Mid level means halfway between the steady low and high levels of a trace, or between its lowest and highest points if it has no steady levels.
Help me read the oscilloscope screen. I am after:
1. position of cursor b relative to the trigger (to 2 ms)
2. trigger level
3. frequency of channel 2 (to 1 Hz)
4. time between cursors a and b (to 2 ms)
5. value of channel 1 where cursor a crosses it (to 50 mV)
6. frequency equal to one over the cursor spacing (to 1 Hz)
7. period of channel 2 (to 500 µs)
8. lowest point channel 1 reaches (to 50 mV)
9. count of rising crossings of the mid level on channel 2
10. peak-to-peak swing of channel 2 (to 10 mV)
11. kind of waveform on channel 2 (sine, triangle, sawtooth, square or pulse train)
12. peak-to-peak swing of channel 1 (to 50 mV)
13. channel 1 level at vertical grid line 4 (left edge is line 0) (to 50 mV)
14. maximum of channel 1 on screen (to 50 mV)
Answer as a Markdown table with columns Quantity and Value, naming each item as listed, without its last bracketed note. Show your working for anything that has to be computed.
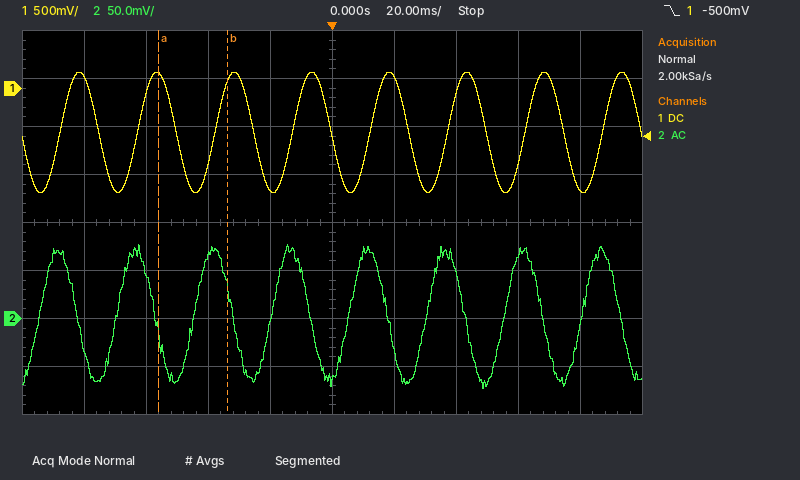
| Quantity | Value |
|---|---|
| position of cursor b relative to the trigger | -34 ms |
| trigger level | -500 mV |
| frequency of channel 2 | 1 / 25.0 ms ≈ 40 Hz |
| time between cursors a and b | 22 ms |
| value of channel 1 where cursor a crosses it | 150 mV |
| frequency equal to one over the cursor spacing | 1 / 22 ms ≈ 45 Hz |
| period of channel 2 | 25.0 ms |
| lowest point channel 1 reaches | -1.10 V |
| count of rising crossings of the mid level on channel 2 | 8 |
| peak-to-peak swing of channel 2 | 150 mV |
| kind of waveform on channel 2 | sine |
| peak-to-peak swing of channel 1 | 150 mV − (-1.10 V) = 1.25 V |
| channel 1 level at vertical grid line 4 (left edge is line 0) | -1.05 V |
| maximum of channel 1 on screen | 150 mV |
